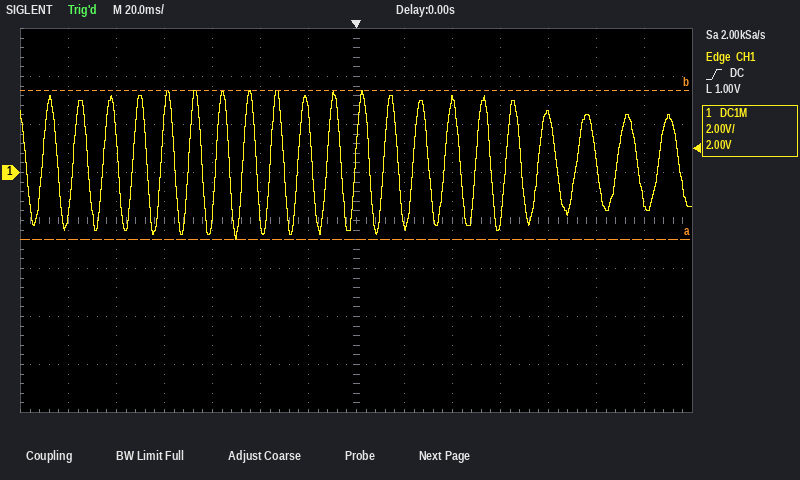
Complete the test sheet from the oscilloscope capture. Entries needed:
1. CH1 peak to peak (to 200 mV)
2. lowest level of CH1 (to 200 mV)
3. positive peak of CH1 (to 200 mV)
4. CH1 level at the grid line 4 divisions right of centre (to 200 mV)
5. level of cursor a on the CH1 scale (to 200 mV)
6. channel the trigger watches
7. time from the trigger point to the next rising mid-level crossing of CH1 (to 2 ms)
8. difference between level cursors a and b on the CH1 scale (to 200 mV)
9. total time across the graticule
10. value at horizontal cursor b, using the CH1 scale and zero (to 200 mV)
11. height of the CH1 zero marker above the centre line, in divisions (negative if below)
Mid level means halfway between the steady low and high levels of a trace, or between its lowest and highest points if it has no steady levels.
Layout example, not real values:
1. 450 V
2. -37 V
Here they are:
1. 6.2 V
2. -2.8 V
3. 3.4 V
4. 2.4 V
5. -2.8 V
6. CH1
7. 12 ms
8. 6.2 V
9. 280 ms
10. 3.4 V
11. +1.0 div
